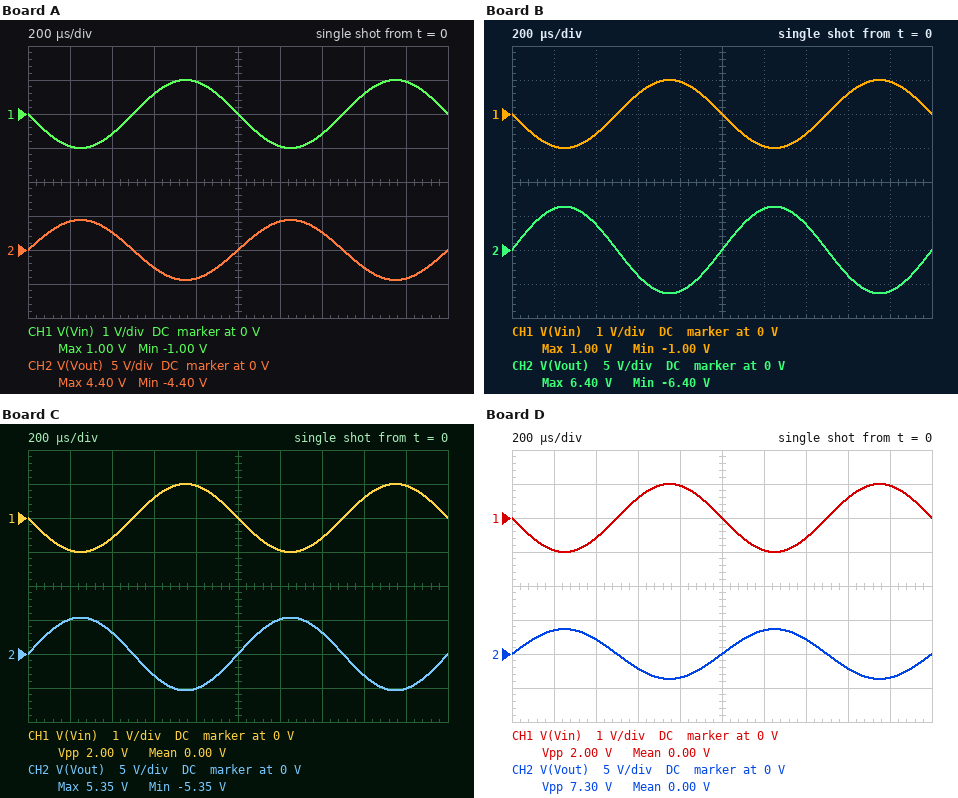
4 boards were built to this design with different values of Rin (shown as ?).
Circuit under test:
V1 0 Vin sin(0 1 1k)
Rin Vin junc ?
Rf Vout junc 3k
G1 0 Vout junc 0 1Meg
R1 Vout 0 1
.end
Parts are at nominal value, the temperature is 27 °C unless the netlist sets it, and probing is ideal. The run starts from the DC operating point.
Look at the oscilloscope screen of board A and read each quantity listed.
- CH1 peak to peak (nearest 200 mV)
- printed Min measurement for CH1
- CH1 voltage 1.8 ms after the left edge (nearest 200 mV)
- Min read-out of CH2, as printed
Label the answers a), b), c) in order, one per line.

a) 2.0 V
b) -1.00 V
c) 1.0 V
d) -4.40 V
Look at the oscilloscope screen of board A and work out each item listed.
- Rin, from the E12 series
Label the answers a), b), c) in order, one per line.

a) 680 Ω
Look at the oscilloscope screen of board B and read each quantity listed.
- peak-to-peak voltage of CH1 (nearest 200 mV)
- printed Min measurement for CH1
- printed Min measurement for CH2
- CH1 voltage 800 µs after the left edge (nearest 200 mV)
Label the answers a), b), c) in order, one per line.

a) 2.0 V
b) -1.00 V
c) -6.40 V
d) 1.0 V
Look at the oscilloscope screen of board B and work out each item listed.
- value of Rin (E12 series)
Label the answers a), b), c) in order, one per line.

a) 470 Ω
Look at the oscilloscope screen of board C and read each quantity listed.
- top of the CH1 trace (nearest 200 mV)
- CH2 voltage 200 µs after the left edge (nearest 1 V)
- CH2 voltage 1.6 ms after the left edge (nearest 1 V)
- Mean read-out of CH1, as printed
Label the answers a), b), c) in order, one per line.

a) 1.0 V
b) 5 V
c) -3 V
d) 0.00 V
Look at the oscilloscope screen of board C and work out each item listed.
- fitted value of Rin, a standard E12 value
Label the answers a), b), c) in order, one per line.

a) 560 Ω
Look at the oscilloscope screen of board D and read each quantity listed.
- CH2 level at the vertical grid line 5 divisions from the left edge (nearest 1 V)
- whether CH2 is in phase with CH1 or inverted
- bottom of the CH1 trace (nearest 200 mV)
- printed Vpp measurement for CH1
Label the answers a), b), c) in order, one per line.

a) 0 V
b) inverted
c) -1.0 V
d) 2.00 V
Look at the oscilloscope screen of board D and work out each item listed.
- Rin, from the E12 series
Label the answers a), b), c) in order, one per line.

a) 820 Ω
